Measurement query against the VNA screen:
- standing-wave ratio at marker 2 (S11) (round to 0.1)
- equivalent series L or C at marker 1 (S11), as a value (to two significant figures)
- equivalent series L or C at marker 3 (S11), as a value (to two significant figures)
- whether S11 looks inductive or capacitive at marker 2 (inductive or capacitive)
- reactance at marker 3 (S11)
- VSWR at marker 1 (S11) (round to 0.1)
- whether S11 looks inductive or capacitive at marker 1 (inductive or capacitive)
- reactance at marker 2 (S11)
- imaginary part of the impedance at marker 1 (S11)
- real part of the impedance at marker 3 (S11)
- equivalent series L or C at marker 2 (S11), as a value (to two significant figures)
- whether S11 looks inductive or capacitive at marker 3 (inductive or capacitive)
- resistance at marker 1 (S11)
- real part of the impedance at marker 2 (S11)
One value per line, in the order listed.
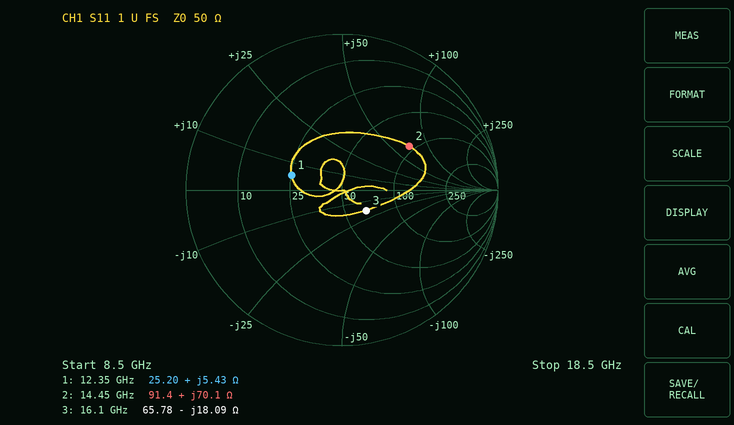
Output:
3.1
70 pH
550 fF
inductive
-18.09 Ω
2.0
inductive
+70.1 Ω
+5.43 Ω
65.78 Ω
770 pH
capacitive
25.20 Ω
91.4 Ω
